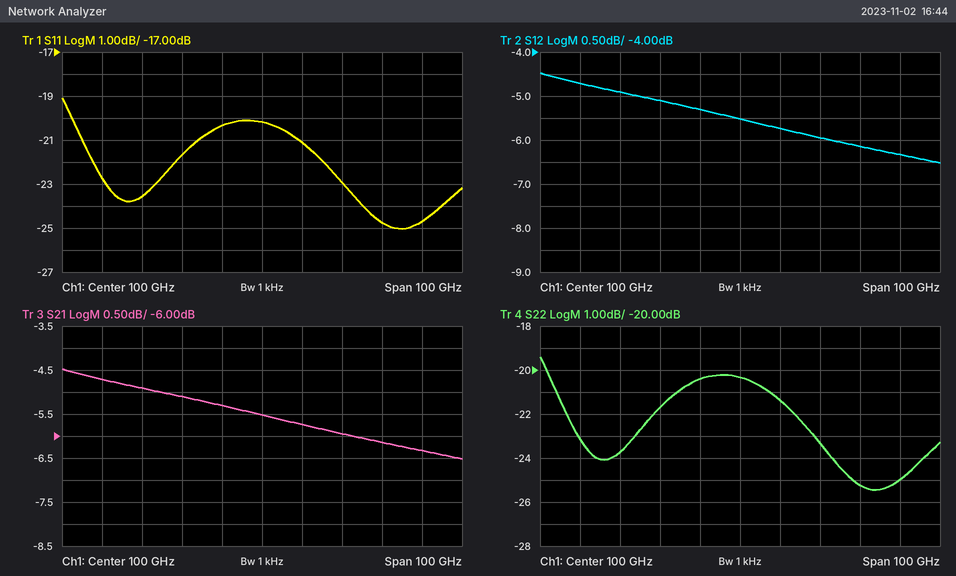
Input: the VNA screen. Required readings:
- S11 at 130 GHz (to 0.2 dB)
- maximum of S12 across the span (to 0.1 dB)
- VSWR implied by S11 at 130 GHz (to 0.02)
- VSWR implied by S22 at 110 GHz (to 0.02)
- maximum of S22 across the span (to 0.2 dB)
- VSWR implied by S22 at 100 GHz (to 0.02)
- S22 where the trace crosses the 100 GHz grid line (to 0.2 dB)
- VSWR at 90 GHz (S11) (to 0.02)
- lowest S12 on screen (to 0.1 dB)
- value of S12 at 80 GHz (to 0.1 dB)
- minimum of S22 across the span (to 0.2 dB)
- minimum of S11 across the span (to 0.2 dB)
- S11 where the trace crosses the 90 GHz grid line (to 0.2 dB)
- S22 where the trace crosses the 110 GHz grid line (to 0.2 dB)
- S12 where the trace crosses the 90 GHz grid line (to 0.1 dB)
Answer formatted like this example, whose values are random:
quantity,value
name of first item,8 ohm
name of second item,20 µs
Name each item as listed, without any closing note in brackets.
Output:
quantity,value
S11 at 130 GHz,-24.8 dB
maximum of S12 across the span,-4.5 dB
VSWR implied by S11 at 130 GHz,1.12
VSWR implied by S22 at 110 GHz,1.18
maximum of S22 across the span,-19.4 dB
VSWR implied by S22 at 100 GHz,1.22
S22 where the trace crosses the 100 GHz grid line,-20.4 dB
VSWR at 90 GHz (S11),1.22
lowest S12 on screen,-6.5 dB
value of S12 at 80 GHz,-5.1 dB
minimum of S22 across the span,-25.4 dB
minimum of S11 across the span,-25.0 dB
S11 where the trace crosses the 90 GHz grid line,-20.4 dB
S22 where the trace crosses the 110 GHz grid line,-21.4 dB
S12 where the trace crosses the 90 GHz grid line,-5.3 dB
